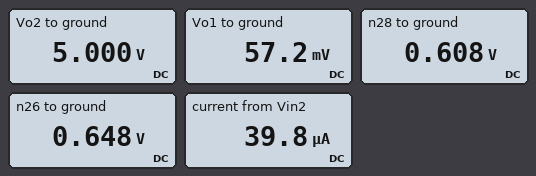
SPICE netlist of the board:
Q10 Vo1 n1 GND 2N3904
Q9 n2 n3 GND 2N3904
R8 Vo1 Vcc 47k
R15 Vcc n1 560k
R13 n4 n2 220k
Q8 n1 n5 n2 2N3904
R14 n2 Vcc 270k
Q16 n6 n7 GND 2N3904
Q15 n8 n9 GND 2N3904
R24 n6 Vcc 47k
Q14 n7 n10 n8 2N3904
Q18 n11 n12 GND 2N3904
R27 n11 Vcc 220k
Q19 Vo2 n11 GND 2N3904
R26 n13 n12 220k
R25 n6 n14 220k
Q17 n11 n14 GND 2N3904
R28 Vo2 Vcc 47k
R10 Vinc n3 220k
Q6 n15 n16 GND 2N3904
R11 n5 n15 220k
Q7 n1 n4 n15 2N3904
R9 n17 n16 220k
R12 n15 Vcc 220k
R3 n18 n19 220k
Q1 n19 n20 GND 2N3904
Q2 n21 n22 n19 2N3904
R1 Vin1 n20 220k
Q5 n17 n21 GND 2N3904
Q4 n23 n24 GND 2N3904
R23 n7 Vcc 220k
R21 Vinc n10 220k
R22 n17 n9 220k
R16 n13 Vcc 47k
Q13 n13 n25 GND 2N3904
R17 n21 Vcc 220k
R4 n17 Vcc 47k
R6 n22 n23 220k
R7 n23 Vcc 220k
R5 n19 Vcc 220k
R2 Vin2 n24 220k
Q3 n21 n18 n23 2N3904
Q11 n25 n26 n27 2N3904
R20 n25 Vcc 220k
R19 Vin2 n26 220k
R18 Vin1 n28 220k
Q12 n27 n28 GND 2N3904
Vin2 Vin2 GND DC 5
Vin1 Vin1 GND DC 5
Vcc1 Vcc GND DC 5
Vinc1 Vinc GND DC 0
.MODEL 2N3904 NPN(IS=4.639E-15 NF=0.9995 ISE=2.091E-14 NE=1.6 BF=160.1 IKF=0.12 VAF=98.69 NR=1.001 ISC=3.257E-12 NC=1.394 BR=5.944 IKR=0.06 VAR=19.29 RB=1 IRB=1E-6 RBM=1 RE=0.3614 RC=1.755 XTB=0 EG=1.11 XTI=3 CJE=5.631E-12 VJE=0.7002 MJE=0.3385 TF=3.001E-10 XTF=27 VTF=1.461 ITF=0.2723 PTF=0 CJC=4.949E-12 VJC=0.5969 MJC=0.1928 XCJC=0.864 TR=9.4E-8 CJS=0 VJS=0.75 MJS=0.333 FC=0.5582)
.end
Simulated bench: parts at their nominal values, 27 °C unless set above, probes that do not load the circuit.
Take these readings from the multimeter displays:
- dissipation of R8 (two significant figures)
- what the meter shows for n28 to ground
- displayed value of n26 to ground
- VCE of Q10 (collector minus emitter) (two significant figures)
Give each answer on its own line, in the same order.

520 µW
0.608 V
0.648 V
57 mV
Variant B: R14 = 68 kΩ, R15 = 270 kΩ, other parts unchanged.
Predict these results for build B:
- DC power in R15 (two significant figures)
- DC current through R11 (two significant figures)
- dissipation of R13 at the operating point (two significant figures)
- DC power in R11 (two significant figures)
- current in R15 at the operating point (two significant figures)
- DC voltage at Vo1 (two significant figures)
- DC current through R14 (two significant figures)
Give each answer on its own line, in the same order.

71 µW
5.5 µA
36 µW
6.6 µW
16 µA
46 mV
15 µA
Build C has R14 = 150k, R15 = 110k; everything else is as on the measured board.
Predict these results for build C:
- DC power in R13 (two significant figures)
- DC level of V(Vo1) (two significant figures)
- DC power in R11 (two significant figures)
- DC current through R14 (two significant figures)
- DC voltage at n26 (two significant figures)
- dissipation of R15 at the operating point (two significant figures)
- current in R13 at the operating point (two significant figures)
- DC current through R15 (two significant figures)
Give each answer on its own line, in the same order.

19 µW
38 mV
9.5 µW
12 µA
650 mV
170 µW
9.2 µA
40 µA
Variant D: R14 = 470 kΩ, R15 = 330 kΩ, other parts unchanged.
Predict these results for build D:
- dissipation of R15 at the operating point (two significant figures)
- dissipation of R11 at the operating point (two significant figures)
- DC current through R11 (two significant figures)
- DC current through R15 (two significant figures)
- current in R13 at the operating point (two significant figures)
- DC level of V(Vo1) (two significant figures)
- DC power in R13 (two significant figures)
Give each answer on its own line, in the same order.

58 µW
15 µW
8.2 µA
13 µA
3.2 µA
55 mV
2.3 µW
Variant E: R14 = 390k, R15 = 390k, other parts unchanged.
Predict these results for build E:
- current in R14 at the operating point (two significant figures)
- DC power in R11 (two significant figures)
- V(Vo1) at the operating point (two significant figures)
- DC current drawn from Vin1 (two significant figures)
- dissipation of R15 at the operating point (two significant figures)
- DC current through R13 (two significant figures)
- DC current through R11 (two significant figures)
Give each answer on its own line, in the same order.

7.6 µA
14 µW
56 mV
40 µA
49 µW
4.1 µA
8.0 µA
